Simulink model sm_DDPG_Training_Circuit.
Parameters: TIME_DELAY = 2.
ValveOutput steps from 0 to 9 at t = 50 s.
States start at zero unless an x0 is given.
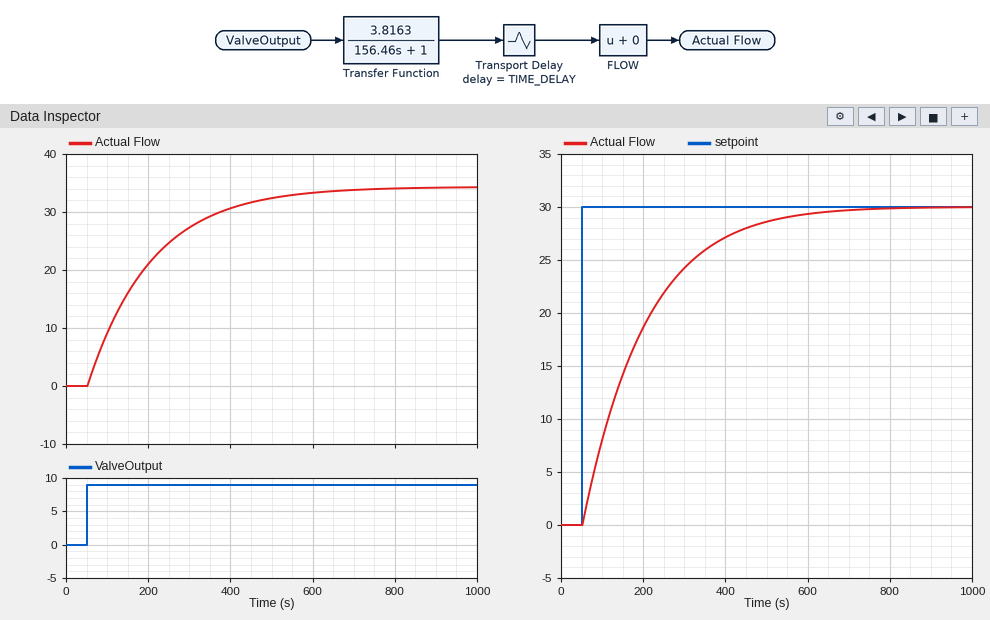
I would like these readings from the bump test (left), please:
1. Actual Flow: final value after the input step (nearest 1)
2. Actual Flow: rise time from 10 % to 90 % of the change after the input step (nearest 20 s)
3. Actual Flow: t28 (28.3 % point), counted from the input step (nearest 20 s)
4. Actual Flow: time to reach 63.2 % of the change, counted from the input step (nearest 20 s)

34
340 s
60 s
160 s
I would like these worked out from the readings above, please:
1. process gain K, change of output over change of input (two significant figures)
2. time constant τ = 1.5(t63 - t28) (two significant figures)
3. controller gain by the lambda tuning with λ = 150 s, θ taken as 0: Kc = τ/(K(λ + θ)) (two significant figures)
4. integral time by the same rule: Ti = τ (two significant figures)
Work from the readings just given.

3.8
150 s
0.26
150 s
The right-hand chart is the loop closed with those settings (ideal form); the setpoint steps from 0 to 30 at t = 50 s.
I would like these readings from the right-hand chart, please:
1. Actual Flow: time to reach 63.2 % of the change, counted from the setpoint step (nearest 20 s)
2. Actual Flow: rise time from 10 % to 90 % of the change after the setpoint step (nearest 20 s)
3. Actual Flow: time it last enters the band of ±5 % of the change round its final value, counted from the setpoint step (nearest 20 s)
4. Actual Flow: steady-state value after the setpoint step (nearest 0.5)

160 s
320 s
440 s
30.0
